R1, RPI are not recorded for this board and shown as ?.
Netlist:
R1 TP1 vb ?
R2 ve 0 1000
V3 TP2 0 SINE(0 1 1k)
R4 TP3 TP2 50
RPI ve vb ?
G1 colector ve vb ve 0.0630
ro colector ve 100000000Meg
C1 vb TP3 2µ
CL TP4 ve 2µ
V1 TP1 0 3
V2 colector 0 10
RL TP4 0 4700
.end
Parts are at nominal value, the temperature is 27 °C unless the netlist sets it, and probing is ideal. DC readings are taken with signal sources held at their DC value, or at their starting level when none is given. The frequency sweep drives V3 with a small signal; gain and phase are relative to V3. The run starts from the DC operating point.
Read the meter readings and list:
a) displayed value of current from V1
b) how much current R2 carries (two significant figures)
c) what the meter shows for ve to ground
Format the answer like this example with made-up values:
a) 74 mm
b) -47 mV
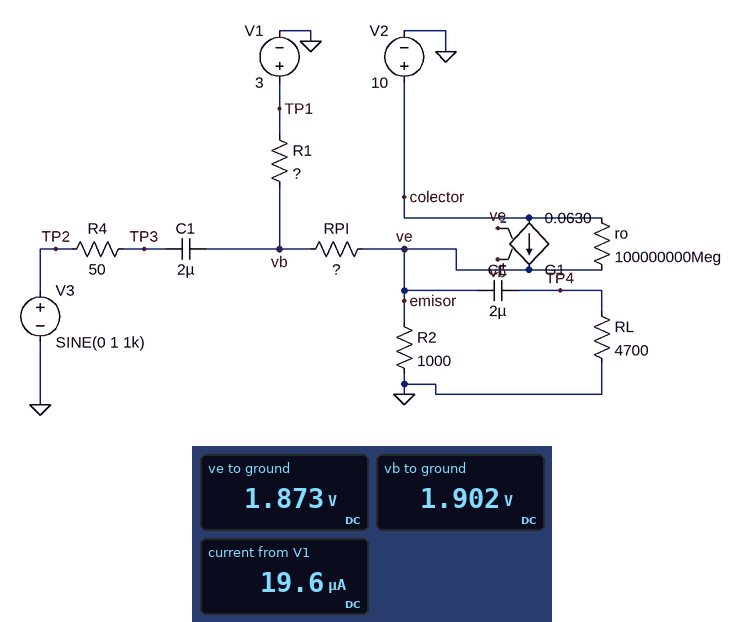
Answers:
a) 19.6 µA
b) 1.9 mA
c) 1.873 V
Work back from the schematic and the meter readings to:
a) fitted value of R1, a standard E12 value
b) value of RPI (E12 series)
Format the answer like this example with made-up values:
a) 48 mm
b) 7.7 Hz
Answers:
a) 56 kΩ
b) 1.5 kΩ
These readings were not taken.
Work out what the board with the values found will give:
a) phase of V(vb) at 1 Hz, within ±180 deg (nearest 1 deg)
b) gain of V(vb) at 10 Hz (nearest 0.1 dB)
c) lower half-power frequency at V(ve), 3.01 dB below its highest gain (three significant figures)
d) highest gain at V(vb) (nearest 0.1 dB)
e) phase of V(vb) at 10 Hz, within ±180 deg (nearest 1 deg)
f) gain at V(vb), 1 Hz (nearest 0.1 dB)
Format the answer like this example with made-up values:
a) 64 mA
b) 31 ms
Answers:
a) 66 deg
b) -0.3 dB
c) 2.25 Hz
d) 0 dB
e) 13 deg
f) -7.8 dB
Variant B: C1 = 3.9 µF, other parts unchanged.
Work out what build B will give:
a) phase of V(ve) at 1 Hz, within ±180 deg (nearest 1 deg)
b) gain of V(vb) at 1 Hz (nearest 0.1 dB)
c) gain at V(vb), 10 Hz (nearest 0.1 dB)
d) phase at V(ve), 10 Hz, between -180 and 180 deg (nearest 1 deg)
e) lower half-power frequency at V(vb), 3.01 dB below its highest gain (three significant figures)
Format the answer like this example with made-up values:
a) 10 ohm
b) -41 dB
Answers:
a) 49 deg
b) -3.7 dB
c) -0.1 dB
d) 7 deg
e) 1.15 Hz
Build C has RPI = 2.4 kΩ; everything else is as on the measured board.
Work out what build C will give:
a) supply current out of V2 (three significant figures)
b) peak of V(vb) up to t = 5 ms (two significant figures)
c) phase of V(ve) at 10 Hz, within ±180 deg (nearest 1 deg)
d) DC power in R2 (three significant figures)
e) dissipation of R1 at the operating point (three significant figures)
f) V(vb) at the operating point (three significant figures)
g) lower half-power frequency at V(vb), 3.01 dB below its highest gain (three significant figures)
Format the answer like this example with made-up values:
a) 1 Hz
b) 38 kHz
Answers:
a) 2.15 mA
b) 3.2 V
c) 11 deg
d) 4.70 mW
e) 11.4 µW
f) 2.20 V
g) 1.95 Hz
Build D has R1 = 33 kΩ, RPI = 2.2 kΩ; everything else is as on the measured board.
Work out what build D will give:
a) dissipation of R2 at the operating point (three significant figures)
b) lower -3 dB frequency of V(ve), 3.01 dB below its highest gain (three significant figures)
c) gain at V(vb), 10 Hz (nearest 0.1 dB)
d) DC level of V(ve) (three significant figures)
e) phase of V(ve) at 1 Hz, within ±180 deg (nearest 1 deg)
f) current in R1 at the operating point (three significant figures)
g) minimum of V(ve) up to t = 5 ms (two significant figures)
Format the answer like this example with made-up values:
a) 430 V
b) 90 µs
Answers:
a) 5.74 mW
b) 2.97 Hz
c) -0.4 dB
d) 2.40 V
e) 71 deg
f) 17.2 µA
g) 1.4 V
